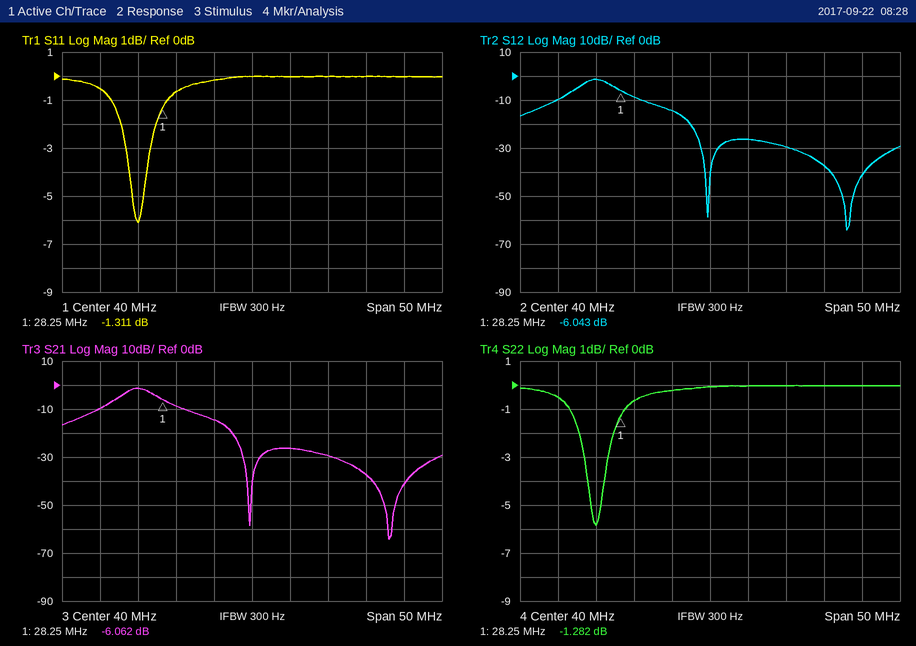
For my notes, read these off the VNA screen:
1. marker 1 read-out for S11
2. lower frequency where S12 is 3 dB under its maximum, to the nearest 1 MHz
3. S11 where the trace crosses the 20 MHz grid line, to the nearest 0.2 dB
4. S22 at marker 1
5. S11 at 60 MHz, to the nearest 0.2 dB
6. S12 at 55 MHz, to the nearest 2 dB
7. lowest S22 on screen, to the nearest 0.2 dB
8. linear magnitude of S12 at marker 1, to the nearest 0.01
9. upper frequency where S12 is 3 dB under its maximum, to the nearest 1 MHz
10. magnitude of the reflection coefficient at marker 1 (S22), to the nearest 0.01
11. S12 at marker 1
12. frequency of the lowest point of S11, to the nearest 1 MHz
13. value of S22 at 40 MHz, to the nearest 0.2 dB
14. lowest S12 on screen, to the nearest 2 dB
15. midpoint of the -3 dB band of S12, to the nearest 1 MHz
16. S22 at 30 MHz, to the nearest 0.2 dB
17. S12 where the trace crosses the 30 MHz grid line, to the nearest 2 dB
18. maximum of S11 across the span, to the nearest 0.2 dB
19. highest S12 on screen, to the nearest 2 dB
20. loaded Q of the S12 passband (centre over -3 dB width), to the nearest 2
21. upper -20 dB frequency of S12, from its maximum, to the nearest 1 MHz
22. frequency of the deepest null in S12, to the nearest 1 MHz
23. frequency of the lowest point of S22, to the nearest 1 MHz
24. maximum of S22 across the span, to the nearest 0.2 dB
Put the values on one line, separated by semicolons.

-1.311 dB; 23 MHz; -0.6 dB; -1.282 dB; 0.0 dB; -38 dB; -5.8 dB; 0.50; 27 MHz; 0.86; -6.043 dB; 25 MHz; 0.0 dB; -64 dB; 25 MHz; -0.6 dB; -8 dB; 0.0 dB; -2 dB; 6; 38 MHz; 58 MHz; 25 MHz; 0.0 dB
